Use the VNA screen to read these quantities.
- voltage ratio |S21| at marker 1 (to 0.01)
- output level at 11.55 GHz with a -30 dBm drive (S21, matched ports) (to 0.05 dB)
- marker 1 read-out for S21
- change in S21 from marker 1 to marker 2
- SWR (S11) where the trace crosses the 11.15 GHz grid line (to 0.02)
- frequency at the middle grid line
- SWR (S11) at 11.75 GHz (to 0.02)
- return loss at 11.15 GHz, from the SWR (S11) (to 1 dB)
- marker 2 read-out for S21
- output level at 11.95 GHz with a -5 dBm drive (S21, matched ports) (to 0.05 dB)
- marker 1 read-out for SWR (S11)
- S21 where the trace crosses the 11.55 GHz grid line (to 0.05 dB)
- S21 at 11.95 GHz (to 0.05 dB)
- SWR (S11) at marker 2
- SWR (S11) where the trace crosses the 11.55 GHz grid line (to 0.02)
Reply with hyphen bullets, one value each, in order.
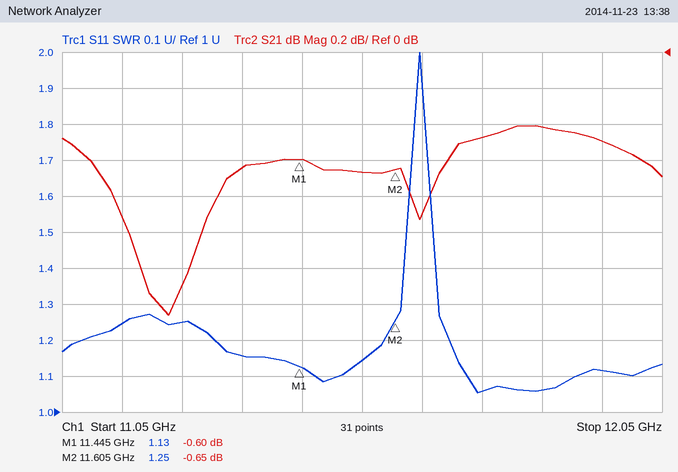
- 0.93
- -30.65 dBm
- -0.60 dB
- -0.05 dB
- 1.24
- 11.55 GHz
- 1.06
- 19 dB
- -0.65 dB
- -5.50 dBm
- 1.13
- -0.65 dB
- -0.50 dB
- 1.25
- 1.14
